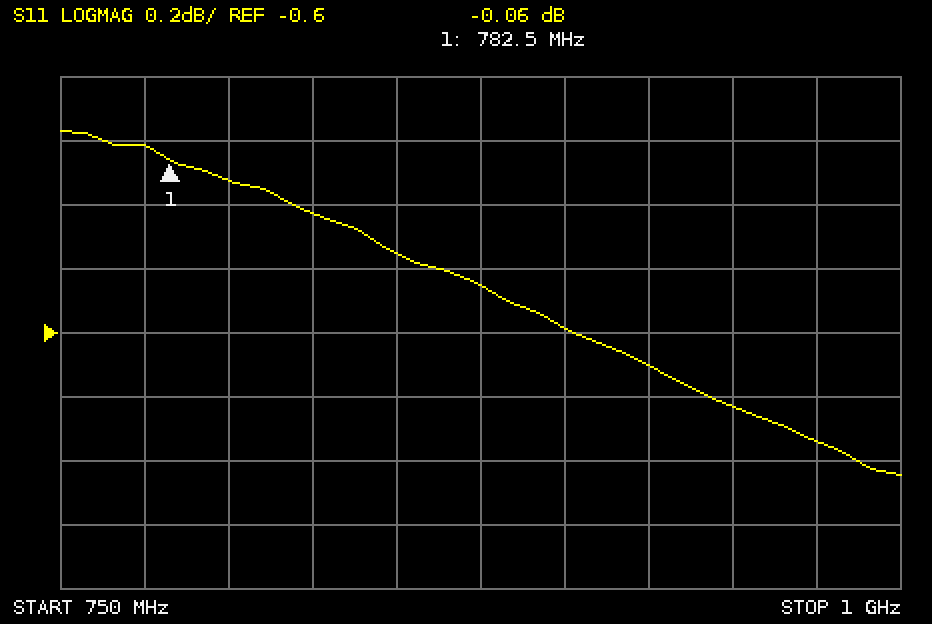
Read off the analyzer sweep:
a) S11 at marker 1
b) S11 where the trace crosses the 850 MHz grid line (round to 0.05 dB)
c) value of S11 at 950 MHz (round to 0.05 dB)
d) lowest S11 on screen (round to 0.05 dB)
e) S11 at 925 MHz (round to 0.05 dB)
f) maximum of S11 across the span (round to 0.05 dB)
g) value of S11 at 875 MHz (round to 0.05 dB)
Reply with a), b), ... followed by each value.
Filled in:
a) -0.06 dB
b) -0.35 dB
c) -0.85 dB
d) -1.05 dB
e) -0.70 dB
f) 0.05 dB
g) -0.45 dB
